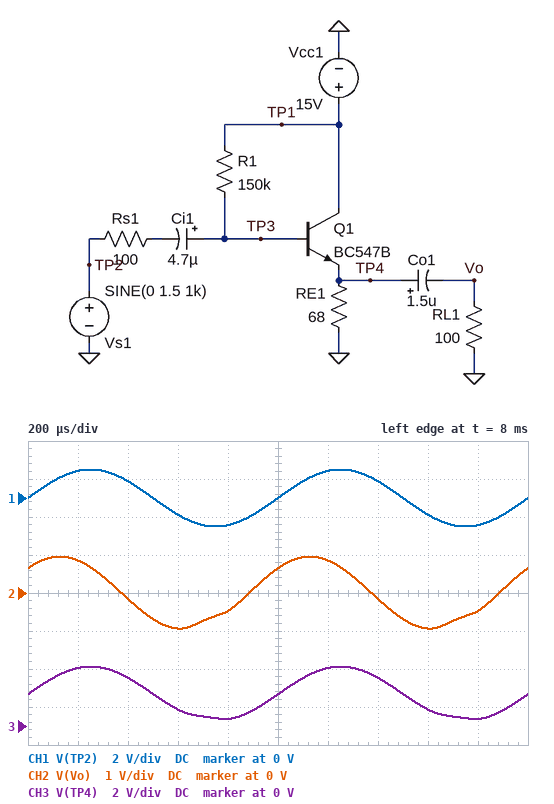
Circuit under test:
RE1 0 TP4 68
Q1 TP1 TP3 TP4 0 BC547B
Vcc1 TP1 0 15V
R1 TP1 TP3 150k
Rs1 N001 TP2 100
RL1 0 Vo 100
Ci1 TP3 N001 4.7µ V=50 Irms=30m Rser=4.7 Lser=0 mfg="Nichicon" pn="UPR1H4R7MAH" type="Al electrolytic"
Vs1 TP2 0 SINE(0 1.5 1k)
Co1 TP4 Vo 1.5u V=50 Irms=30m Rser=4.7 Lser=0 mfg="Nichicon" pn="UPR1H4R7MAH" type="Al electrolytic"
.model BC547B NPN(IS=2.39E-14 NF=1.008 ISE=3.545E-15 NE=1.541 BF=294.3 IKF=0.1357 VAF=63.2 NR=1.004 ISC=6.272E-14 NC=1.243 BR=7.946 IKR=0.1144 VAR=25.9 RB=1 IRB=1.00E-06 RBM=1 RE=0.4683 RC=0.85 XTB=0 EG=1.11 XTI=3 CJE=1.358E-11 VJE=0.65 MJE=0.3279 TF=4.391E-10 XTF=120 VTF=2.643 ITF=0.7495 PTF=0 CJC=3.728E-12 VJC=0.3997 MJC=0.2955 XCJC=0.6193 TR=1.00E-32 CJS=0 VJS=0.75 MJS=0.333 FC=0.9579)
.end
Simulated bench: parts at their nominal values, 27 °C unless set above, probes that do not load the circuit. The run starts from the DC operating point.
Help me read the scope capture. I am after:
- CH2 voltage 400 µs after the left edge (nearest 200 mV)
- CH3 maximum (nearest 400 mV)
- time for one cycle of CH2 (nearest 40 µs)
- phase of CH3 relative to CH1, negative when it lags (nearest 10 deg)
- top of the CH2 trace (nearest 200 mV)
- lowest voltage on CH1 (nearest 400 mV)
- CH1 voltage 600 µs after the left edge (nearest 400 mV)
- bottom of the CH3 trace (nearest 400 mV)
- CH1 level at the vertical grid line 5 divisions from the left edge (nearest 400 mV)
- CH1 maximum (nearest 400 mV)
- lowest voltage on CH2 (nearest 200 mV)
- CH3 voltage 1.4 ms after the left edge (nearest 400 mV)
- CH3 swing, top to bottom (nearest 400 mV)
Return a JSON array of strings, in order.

["-200 mV", "3.2 V", "1.00 ms", "0 deg", "1.0 V", "-1.6 V", "-800 mV", "400 mV", "0 V", "1.6 V", "-1.0 V", "2.4 V", "2.8 V"]
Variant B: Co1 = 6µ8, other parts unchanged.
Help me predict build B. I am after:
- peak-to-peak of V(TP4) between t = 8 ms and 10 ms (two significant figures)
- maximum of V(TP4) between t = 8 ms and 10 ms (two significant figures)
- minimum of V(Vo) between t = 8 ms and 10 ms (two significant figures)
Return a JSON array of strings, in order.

["2.5 V", "3.1 V", "-1.1 V"]
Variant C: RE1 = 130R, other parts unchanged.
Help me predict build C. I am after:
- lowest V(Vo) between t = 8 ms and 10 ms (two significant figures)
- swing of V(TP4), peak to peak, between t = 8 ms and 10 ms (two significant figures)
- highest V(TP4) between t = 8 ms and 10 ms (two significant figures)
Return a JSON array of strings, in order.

["-970 mV", "2.9 V", "4.4 V"]
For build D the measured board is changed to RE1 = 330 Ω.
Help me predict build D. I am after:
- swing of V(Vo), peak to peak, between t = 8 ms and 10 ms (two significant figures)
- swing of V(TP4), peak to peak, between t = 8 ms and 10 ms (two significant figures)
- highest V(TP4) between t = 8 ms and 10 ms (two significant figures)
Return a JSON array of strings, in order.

["2.0 V", "2.9 V", "7.1 V"]
